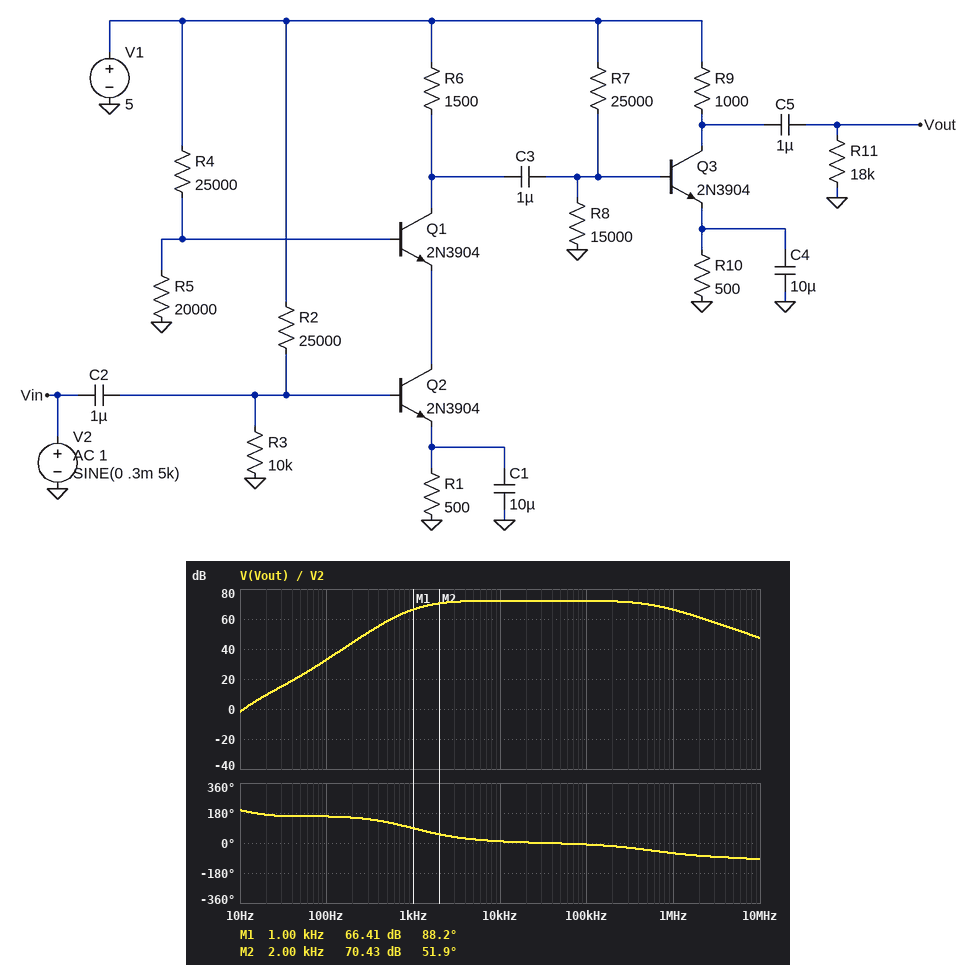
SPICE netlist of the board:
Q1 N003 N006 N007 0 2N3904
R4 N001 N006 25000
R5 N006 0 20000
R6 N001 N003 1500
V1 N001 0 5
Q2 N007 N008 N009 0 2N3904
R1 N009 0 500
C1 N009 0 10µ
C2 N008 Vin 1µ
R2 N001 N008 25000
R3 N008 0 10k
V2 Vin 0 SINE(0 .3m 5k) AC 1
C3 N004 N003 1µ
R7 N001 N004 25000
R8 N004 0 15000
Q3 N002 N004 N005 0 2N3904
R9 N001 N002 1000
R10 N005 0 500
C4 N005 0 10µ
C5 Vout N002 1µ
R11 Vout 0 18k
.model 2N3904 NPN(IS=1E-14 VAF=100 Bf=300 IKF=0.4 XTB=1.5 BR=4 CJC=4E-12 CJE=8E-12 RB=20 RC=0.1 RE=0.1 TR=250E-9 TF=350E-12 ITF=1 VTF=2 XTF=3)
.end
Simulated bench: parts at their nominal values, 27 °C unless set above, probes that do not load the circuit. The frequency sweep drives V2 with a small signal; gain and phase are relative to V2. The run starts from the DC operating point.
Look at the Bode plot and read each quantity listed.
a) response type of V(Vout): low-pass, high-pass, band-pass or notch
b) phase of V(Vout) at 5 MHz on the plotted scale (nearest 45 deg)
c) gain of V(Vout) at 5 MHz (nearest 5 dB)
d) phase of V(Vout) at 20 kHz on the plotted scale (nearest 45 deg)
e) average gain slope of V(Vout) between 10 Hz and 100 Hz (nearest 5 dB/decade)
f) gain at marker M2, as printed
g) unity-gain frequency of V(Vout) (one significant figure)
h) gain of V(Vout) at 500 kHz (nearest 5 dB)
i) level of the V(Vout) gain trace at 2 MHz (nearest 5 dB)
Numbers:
band-pass
-90 deg
55 dB
0 deg
35 dB/decade
70.43 dB
10 Hz
70 dB
60 dB
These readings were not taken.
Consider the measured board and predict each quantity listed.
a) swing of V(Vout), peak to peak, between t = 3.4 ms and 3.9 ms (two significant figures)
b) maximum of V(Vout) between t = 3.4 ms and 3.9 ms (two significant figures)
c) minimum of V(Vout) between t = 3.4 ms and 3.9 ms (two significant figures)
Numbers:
2.3 V
1.0 V
-1.3 V
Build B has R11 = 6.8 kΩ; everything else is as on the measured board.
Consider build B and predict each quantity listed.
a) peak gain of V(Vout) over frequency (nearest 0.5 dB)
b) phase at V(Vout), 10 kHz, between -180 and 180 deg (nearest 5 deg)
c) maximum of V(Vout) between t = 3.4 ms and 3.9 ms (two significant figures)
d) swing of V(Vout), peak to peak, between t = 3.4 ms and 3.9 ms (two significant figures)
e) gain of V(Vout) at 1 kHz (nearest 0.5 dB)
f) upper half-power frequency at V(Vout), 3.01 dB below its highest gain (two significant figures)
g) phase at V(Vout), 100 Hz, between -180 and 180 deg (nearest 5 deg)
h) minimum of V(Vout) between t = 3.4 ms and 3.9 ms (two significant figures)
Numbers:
71.5 dB
10 deg
960 mV
2.1 V
65.5 dB
610 kHz
165 deg
-1.2 V
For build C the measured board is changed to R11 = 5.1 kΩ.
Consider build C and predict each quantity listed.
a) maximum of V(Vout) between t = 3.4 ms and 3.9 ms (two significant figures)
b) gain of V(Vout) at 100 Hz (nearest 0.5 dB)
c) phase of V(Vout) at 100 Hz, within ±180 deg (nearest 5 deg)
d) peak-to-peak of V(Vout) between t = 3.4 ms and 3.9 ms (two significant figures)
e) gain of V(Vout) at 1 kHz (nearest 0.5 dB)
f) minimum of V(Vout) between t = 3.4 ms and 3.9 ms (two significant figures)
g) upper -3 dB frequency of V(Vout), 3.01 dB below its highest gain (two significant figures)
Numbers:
920 mV
31.5 dB
170 deg
2.0 V
65.5 dB
-1.1 V
630 kHz
